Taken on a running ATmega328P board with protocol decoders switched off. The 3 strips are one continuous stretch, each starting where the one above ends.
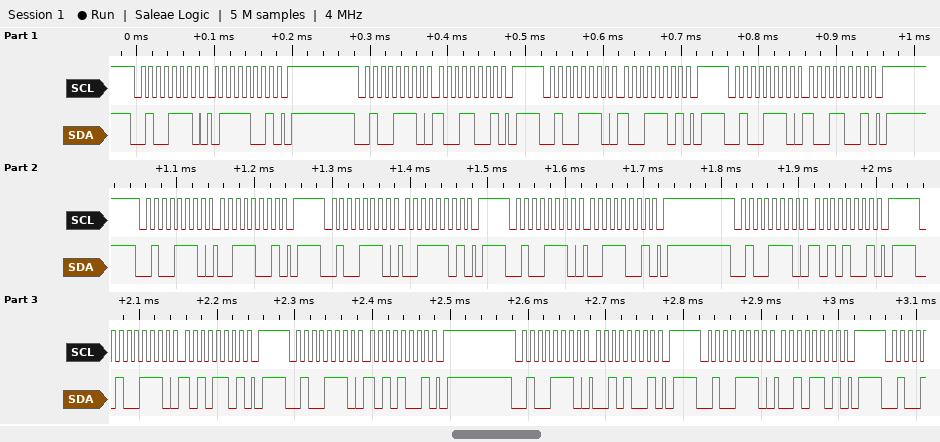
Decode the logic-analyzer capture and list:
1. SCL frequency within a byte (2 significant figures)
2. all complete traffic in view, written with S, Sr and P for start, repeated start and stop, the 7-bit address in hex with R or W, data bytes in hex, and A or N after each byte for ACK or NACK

100 kHz
S 27W A 79 A P S 27W A 99 A P S 27W A 9D A P S 27W A 99 A P S 27W A 39 A P S 27W A 3D A P S 27W A 39 A P S 27W A A9 A P S 27W A AD A P S 27W A A9 A P S 27W A 29 A P S 27W A 2D A P
